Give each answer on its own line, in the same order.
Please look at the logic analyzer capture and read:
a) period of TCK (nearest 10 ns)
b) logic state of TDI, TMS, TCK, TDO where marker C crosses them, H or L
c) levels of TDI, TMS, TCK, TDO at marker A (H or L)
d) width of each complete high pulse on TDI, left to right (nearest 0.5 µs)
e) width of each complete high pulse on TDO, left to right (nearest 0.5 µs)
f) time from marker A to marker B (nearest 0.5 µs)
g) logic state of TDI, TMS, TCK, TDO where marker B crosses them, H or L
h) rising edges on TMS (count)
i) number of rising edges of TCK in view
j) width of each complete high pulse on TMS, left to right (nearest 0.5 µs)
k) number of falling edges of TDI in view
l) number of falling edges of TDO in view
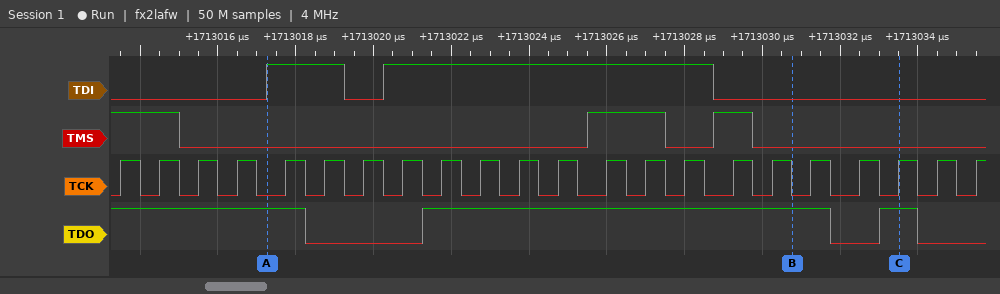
1050 ns
TDI=L, TMS=L, TCK=H, TDO=H
TDI=H, TMS=L, TCK=L, TDO=H
2 µs, 8.5 µs
10.5 µs, 1 µs
13.5 µs
TDI=L, TMS=L, TCK=L, TDO=H
2
22
2 µs, 1 µs
2
3
